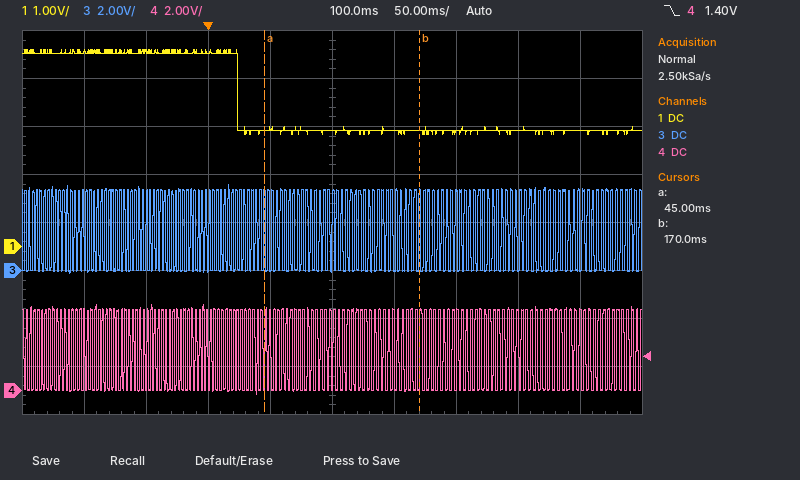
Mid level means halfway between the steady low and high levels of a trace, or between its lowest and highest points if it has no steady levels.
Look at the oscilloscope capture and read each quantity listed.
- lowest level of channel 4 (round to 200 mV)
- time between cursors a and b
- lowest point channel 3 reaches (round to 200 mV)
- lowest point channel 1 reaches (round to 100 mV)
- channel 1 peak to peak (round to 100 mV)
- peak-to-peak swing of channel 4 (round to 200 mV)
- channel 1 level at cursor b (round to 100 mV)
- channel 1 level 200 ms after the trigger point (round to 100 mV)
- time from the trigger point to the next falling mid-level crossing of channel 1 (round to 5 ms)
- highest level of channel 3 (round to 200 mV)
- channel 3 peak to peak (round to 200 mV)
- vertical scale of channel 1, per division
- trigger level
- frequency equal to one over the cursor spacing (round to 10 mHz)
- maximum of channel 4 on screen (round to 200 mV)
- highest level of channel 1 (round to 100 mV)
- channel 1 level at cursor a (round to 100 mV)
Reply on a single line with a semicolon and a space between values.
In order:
-200 mV; 125 ms; -200 mV; 2.3 V; 1.8 V; 3.8 V; 2.4 V; 2.4 V; 25 ms; 3.6 V; 3.8 V; 1 V; 1.40 V; 8.00 Hz; 3.6 V; 4.1 V; 2.4 V
